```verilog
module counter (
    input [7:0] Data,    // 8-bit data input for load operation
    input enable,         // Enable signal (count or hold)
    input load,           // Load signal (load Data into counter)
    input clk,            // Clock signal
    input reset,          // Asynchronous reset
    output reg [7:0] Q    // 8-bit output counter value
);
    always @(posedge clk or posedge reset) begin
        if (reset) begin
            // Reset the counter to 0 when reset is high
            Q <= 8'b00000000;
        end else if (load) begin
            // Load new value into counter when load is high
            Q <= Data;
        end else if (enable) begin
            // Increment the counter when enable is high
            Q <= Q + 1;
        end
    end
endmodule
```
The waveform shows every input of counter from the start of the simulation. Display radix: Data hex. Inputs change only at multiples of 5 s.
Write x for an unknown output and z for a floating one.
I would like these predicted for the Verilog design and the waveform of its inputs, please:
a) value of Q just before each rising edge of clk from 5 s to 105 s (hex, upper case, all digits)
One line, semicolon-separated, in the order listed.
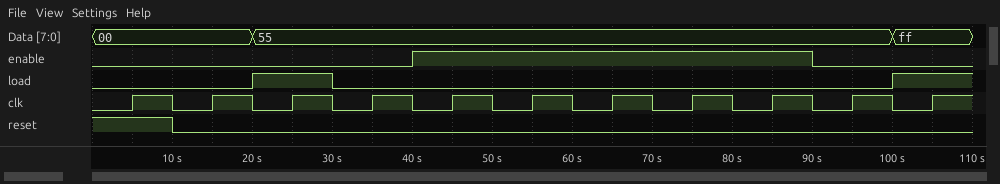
00, 00, 00, 55, 55, 56, 57, 58, 59, 5A, 5A
